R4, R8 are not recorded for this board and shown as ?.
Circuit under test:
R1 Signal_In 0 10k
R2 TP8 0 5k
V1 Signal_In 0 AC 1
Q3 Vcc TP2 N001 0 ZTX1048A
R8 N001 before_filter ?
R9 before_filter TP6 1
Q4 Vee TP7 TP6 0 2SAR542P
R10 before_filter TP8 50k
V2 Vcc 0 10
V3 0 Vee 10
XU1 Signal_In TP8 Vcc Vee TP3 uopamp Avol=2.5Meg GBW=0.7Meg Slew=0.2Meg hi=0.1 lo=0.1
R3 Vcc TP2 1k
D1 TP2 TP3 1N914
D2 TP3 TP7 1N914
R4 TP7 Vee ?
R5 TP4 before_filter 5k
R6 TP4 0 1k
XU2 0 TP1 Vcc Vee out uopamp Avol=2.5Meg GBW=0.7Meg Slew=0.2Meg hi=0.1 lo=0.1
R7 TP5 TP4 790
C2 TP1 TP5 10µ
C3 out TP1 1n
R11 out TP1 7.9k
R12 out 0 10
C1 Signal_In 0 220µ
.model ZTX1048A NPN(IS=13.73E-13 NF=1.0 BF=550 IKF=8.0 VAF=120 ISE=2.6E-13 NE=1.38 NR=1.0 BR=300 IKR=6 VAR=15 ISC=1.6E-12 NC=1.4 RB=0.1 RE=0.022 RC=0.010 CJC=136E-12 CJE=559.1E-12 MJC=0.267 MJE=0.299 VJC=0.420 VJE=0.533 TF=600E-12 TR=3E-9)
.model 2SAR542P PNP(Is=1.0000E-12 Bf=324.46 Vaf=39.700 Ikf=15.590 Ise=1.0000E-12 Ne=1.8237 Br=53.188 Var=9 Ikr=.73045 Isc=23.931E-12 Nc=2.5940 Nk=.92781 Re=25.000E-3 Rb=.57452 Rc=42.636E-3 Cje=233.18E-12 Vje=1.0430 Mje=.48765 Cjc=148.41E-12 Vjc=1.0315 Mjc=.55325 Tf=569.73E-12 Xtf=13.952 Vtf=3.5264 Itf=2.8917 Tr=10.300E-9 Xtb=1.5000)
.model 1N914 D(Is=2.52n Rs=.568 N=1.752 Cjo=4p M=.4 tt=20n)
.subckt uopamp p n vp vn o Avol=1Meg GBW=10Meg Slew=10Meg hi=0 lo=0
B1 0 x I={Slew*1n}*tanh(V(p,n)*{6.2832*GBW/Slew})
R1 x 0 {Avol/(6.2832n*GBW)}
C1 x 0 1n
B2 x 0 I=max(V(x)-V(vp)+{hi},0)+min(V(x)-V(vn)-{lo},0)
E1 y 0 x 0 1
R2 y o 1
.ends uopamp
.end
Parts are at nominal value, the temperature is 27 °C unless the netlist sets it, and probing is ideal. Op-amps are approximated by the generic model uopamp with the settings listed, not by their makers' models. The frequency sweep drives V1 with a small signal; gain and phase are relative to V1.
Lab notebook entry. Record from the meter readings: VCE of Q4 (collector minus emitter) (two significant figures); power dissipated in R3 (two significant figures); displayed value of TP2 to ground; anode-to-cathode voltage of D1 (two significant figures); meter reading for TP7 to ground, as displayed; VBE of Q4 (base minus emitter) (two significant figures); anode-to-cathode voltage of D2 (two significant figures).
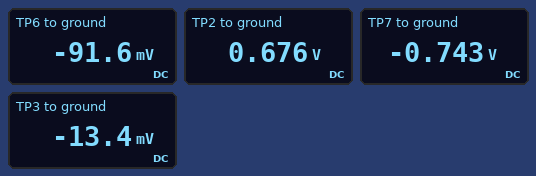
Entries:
-9.9 V
87 mW
0.676 V
690 mV
-0.743 V
-650 mV
730 mV
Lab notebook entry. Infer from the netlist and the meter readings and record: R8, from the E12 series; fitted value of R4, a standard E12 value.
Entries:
0.33 Ω
470 Ω
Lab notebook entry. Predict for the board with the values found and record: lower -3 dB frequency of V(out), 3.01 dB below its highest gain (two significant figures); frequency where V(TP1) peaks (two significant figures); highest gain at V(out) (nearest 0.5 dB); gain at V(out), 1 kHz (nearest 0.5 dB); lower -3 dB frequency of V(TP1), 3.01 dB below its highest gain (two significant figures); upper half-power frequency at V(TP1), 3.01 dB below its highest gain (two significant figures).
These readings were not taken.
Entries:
9.8 Hz
33 kHz
19.0 dB
19.0 dB
12 kHz
91 kHz
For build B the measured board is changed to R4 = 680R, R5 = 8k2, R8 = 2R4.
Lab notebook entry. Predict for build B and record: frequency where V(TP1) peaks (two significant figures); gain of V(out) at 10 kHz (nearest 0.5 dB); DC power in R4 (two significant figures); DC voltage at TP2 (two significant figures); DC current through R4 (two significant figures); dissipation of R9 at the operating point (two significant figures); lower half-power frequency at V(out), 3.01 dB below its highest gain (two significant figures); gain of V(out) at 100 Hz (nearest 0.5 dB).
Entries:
33 kHz
13.5 dB
130 mW
730 mV
14 mA
1.8 mW
9.5 Hz
15.0 dB
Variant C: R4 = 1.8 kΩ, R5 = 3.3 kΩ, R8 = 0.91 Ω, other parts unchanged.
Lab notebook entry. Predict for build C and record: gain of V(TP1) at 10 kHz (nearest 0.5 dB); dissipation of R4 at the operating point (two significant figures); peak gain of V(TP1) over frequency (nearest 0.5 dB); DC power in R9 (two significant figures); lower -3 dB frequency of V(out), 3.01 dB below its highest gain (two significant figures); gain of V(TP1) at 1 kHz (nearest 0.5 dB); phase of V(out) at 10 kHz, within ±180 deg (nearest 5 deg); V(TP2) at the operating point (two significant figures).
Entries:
-15.0 dB
48 mW
-11.0 dB
2.2 mW
10 Hz
-34.0 dB
140 deg
670 mV
